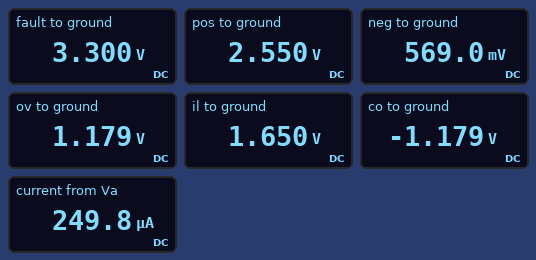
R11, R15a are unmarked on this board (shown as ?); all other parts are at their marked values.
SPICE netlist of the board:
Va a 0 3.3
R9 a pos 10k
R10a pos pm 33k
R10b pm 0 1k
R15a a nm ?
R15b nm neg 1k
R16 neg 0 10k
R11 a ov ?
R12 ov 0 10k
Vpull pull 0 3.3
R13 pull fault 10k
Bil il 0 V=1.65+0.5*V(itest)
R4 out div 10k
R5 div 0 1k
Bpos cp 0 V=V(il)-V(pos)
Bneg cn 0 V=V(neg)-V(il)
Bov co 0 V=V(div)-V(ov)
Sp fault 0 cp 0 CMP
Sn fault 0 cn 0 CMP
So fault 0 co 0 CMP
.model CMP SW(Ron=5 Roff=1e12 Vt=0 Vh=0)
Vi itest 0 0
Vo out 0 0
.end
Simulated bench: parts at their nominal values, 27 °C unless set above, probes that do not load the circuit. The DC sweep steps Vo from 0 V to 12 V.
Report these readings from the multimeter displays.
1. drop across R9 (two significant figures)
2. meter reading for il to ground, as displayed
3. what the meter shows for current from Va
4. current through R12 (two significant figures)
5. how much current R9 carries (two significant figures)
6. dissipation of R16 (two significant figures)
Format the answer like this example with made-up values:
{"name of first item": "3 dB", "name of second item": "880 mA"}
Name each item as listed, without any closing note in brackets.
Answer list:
{"drop across R9": "750 mV", "meter reading for il to ground, as displayed": "1.650 V", "what the meter shows for current from Va": "249.8 µA", "current through R12": "120 µA", "how much current R9 carries": "75 µA", "dissipation of R16": "32 µW"}
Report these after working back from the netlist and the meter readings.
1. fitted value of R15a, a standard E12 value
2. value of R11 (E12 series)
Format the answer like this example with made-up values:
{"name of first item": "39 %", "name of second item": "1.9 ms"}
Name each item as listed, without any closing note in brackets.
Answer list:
{"fitted value of R15a, a standard E12 value": "47 kΩ", "value of R11": "18 kΩ"}
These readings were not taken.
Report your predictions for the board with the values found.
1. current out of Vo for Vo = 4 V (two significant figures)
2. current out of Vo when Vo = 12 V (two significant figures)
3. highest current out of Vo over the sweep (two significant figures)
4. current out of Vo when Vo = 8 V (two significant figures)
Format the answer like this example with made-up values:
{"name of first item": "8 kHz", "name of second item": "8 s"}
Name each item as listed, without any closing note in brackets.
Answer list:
{"current out of Vo for Vo = 4 V": "360 µA", "current out of Vo when Vo = 12 V": "1.1 mA", "highest current out of Vo over the sweep": "1.1 mA", "current out of Vo when Vo = 8 V": "730 µA"}
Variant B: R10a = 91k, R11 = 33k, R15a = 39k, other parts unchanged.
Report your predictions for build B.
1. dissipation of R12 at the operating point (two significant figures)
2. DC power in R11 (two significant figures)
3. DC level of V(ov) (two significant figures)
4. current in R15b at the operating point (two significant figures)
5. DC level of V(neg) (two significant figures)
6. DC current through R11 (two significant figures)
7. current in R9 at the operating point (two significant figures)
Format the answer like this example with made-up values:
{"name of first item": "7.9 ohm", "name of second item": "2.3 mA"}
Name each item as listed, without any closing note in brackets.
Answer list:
{"dissipation of R12 at the operating point": "59 µW", "DC power in R11": "190 µW", "DC level of V(ov)": "770 mV", "current in R15b at the operating point": "66 µA", "DC level of V(neg)": "660 mV", "DC current through R11": "77 µA", "current in R9 at the operating point": "32 µA"}
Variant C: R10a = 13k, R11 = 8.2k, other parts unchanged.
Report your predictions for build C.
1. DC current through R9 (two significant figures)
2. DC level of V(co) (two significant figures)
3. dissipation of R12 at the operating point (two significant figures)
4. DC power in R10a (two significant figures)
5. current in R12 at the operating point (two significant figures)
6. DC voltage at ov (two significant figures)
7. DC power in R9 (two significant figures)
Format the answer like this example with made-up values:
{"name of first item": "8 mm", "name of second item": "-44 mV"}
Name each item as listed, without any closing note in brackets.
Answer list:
{"DC current through R9": "140 µA", "DC level of V(co)": "-1.8 V", "dissipation of R12 at the operating point": "330 µW", "DC power in R10a": "250 µW", "current in R12 at the operating point": "180 µA", "DC voltage at ov": "1.8 V", "DC power in R9": "190 µW"}
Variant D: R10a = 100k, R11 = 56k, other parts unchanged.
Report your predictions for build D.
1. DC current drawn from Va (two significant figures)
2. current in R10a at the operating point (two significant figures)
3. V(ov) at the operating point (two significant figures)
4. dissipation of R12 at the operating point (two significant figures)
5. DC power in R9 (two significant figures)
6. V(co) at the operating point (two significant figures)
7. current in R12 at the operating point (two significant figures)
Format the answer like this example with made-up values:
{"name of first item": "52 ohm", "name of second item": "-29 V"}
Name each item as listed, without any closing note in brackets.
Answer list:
{"DC current drawn from Va": "140 µA", "current in R10a at the operating point": "30 µA", "V(ov) at the operating point": "500 mV", "dissipation of R12 at the operating point": "25 µW", "DC power in R9": "8.8 µW", "V(co) at the operating point": "-500 mV", "current in R12 at the operating point": "50 µA"}
